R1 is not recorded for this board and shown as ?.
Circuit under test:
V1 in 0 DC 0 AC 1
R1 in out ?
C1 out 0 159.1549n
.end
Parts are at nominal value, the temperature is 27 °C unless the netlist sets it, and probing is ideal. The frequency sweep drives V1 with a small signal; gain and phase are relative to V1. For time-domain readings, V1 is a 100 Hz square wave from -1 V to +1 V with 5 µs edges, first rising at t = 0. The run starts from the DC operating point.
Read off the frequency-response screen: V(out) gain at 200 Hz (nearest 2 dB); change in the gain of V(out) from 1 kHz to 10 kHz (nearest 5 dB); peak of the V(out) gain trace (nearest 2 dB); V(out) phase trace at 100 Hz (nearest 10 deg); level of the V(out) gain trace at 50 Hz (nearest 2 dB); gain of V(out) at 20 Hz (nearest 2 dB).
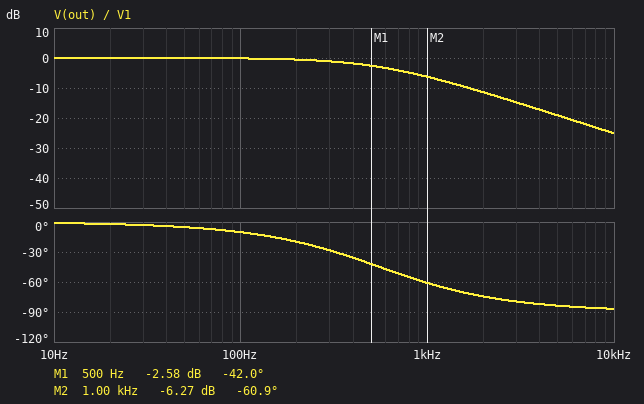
0 dB
-20 dB
0 dB
-10 deg
0 dB
0 dB
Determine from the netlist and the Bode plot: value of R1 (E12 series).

1.8 kΩ
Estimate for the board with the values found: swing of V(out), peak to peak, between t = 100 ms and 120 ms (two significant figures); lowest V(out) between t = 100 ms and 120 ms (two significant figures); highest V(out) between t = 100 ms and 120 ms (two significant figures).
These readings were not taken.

2.0 V
-1.0 V
1.0 V
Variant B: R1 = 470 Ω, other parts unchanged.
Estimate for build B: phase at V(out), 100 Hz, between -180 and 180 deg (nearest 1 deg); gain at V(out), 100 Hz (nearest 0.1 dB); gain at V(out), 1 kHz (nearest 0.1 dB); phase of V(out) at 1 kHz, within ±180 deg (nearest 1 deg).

-3 deg
0 dB
-0.9 dB
-25 deg
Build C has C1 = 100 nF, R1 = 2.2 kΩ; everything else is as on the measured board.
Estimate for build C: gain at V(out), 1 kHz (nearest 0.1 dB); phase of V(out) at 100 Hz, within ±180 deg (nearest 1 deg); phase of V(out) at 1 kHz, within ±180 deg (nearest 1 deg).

-4.6 dB
-8 deg
-54 deg
